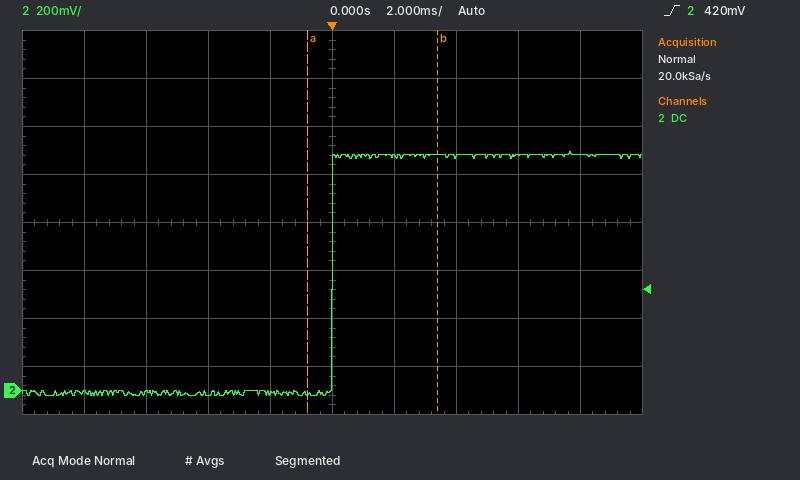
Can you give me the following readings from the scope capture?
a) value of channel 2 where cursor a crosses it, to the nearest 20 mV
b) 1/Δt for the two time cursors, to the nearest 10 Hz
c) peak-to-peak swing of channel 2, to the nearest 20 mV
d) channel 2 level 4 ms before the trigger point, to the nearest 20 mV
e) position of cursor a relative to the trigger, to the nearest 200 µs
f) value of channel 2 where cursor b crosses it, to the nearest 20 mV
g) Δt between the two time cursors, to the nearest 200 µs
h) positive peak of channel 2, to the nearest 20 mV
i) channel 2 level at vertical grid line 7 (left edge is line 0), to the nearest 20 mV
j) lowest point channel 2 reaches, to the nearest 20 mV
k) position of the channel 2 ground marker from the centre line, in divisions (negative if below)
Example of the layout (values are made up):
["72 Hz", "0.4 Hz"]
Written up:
["-20 mV", "240 Hz", "1.02 V", "-20 mV", "-800 µs", "980 mV", "4.2 ms", "1.00 V", "980 mV", "-20 mV", "-3.5 div"]
